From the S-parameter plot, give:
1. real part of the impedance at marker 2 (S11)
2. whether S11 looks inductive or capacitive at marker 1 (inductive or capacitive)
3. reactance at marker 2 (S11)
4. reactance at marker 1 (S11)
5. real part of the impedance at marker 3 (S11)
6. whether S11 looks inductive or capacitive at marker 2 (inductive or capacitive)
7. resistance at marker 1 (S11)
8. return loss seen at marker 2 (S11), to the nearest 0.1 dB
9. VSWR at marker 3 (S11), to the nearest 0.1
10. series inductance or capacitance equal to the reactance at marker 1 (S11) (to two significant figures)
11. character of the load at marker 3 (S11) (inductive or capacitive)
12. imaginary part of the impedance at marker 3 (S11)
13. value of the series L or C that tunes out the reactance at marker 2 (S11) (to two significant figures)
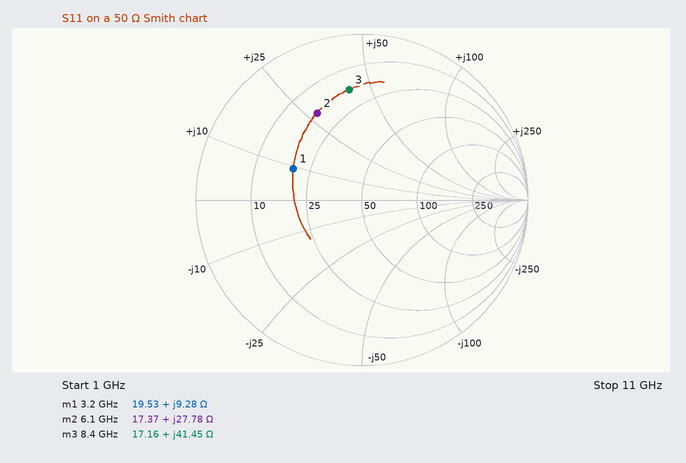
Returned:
17.37 Ω
inductive
+27.78 Ω
+9.28 Ω
17.16 Ω
inductive
19.53 Ω
4.6 dB
5.1
460 pH
inductive
+41.45 Ω
940 fF
